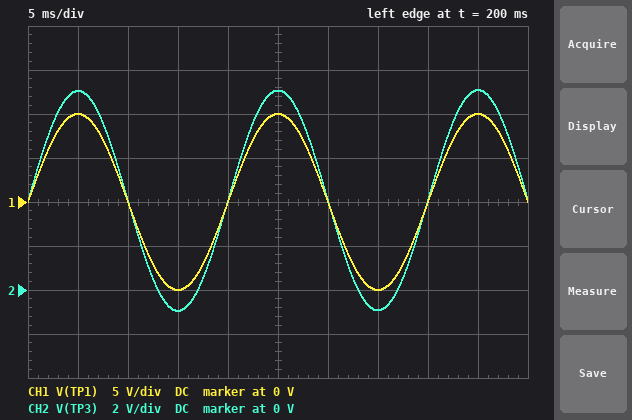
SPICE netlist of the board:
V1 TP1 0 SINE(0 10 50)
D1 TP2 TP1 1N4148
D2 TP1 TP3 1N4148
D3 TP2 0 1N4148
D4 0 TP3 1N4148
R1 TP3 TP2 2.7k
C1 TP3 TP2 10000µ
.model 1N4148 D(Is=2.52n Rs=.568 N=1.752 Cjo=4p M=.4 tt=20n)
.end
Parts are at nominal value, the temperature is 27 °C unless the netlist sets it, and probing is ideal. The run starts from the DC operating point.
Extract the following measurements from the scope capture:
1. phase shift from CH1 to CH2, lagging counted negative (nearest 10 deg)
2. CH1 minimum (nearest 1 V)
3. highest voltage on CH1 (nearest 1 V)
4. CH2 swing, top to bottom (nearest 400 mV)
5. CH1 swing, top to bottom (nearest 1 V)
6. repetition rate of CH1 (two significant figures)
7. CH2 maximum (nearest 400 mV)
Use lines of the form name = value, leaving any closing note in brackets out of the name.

phase shift from CH1 to CH2, lagging counted negative = 0 deg
CH1 minimum = -10 V
highest voltage on CH1 = 10 V
CH2 swing, top to bottom = 10.0 V
CH1 swing, top to bottom = 20 V
repetition rate of CH1 = 50 Hz
CH2 maximum = 9.2 V
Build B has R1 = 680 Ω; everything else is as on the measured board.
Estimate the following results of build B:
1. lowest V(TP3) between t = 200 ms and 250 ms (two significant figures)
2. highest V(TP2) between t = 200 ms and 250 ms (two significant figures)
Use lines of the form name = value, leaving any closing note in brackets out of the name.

lowest V(TP3) between t = 200 ms and 250 ms = -970 mV
highest V(TP2) between t = 200 ms and 250 ms = 980 mV
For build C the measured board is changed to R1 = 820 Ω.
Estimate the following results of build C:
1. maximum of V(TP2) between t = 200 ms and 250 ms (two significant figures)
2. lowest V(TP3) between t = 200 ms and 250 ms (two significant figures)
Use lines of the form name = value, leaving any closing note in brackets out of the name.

maximum of V(TP2) between t = 200 ms and 250 ms = 980 mV
lowest V(TP3) between t = 200 ms and 250 ms = -970 mV
